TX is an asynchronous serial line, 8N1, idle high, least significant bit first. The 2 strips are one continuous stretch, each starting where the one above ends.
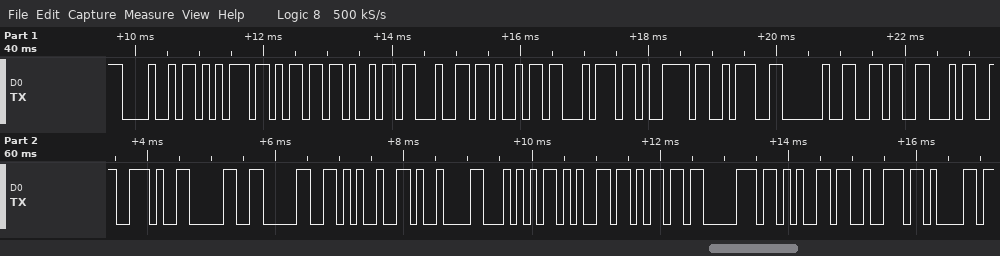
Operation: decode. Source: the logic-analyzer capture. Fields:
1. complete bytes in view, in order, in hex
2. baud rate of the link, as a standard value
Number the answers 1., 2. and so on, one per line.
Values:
1. 48 75 6D 69 64 69 74 79 3A 20 36 34 2E 30 30 25 09 54 65 6D 70 65 72 61
2. 9600 baud
